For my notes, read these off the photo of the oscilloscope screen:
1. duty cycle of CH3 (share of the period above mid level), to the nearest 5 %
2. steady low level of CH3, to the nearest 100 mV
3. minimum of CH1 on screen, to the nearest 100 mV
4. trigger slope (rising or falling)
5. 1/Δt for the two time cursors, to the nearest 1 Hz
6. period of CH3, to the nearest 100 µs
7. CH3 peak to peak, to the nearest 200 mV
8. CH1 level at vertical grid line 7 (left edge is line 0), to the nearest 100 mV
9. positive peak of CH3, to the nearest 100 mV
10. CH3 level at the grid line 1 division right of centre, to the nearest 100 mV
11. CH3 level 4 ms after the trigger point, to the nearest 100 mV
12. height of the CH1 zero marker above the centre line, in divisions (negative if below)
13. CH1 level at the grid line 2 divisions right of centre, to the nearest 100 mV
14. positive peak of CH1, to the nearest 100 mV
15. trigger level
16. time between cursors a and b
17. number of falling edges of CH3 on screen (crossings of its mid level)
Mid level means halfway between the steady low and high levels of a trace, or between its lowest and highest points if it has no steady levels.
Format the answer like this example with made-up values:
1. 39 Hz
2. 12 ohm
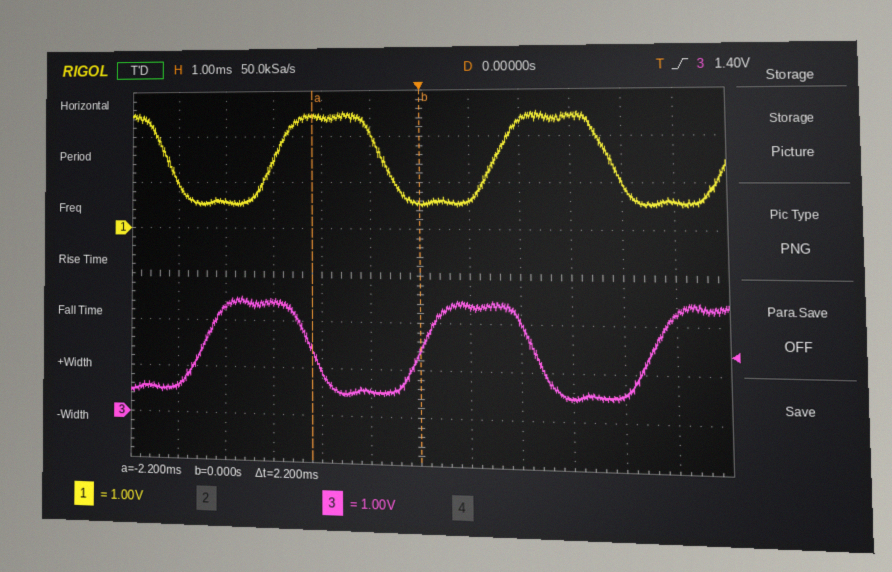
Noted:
1. 50 %
2. 500 mV
3. 500 mV
4. rising
5. 455 Hz
6. 4.5 ms
7. 2.0 V
8. 600 mV
9. 2.5 V
10. 2.4 V
11. 600 mV
12. +1.0 div
13. 2.4 V
14. 2.5 V
15. 1.40 V
16. 2.2 ms
17. 2
